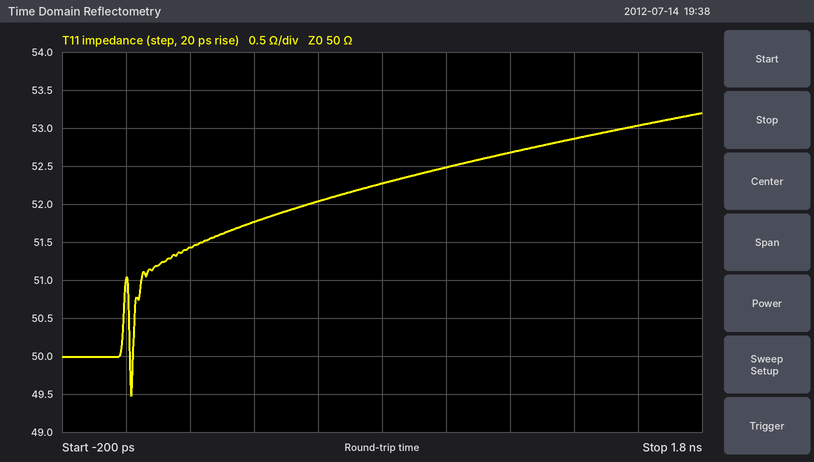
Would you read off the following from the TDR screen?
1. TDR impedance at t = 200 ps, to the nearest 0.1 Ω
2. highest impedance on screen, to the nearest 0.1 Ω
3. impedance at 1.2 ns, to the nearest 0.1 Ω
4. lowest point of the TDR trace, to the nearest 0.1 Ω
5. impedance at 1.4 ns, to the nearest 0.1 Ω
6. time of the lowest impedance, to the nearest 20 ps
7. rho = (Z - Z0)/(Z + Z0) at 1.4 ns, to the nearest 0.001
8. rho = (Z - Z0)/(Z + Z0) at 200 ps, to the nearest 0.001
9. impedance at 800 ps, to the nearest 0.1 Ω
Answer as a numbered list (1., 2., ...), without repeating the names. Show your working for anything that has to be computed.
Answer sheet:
1. 51.4 Ω
2. 53.2 Ω
3. 52.7 Ω
4. 49.5 Ω
5. 52.9 Ω
6. 20 ps
7. (52.9 − 50)/(52.9 + 50) ≈ +0.028
8. (51.4 − 50)/(51.4 + 50) ≈ +0.014
9. 52.3 Ω
